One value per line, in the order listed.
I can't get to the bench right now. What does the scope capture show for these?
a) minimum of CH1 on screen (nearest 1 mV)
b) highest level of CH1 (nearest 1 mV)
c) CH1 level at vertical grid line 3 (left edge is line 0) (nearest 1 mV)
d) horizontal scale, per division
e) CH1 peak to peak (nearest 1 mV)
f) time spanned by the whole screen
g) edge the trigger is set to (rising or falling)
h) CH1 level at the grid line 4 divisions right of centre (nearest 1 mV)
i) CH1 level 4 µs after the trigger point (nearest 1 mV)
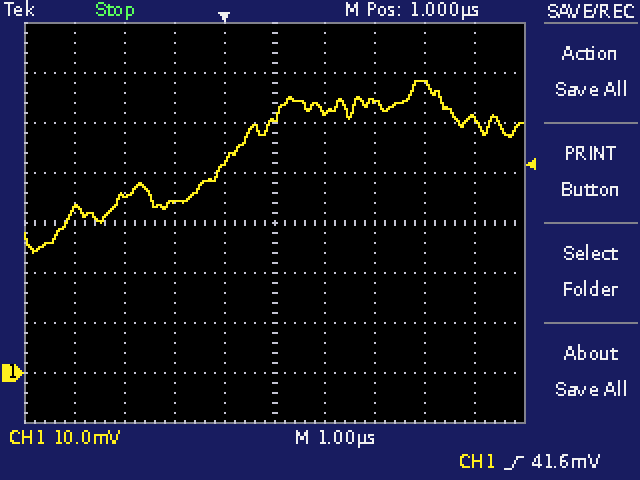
24 mV
58 mV
34 mV
1 µs
34 mV
10 µs
rising
51 mV
58 mV
